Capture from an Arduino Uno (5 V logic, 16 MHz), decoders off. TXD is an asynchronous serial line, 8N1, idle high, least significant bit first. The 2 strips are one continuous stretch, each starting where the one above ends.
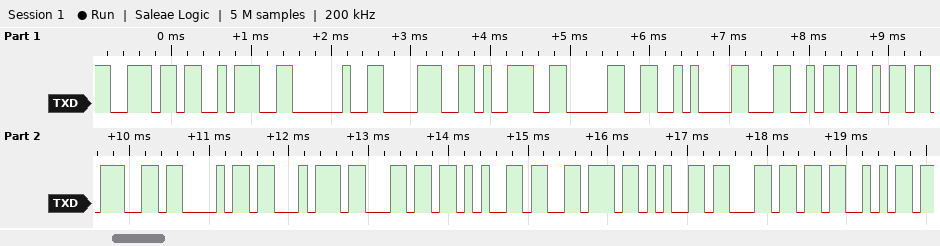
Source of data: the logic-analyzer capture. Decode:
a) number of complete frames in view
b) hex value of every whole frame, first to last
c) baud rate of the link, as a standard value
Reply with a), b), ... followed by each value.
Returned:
a) 18
b) 0x6E 0x3A 0x20 0x38 0x39 0x30 0x0A 0x4C 0x69 0x67 0x68 0x74 0x6C 0x65 0x76 0x65 0x6C 0x53
c) 9600 baud
